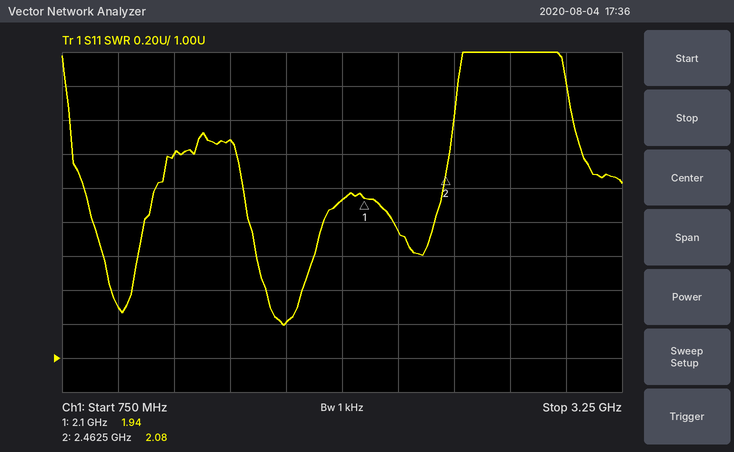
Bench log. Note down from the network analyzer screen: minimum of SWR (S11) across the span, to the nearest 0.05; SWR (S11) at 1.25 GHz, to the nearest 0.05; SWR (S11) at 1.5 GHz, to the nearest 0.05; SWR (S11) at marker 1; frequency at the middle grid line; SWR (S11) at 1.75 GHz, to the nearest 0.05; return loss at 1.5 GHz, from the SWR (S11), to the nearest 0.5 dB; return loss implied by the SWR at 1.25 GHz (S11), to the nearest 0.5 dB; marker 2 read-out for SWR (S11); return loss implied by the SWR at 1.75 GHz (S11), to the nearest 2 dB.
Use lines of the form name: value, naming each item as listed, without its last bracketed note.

minimum of SWR (S11) across the span, to the nearest 0.05: 1.20
SWR (S11) at 1.25 GHz, to the nearest 0.05: 2.20
SWR (S11) at 1.5 GHz, to the nearest 0.05: 2.30
SWR (S11) at marker 1: 1.94
frequency at the middle grid line: 2 GHz
SWR (S11) at 1.75 GHz, to the nearest 0.05: 1.20
return loss at 1.5 GHz, from the SWR (S11), to the nearest 0.5 dB: 8.0 dB
return loss implied by the SWR at 1.25 GHz (S11), to the nearest 0.5 dB: 8.5 dB
marker 2 read-out for SWR: 2.08
return loss implied by the SWR at 1.75 GHz (S11), to the nearest 2 dB: 20 dB
